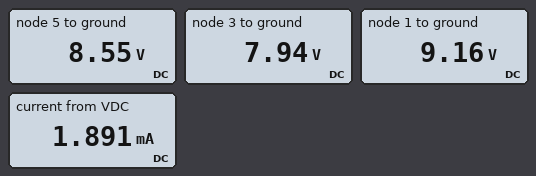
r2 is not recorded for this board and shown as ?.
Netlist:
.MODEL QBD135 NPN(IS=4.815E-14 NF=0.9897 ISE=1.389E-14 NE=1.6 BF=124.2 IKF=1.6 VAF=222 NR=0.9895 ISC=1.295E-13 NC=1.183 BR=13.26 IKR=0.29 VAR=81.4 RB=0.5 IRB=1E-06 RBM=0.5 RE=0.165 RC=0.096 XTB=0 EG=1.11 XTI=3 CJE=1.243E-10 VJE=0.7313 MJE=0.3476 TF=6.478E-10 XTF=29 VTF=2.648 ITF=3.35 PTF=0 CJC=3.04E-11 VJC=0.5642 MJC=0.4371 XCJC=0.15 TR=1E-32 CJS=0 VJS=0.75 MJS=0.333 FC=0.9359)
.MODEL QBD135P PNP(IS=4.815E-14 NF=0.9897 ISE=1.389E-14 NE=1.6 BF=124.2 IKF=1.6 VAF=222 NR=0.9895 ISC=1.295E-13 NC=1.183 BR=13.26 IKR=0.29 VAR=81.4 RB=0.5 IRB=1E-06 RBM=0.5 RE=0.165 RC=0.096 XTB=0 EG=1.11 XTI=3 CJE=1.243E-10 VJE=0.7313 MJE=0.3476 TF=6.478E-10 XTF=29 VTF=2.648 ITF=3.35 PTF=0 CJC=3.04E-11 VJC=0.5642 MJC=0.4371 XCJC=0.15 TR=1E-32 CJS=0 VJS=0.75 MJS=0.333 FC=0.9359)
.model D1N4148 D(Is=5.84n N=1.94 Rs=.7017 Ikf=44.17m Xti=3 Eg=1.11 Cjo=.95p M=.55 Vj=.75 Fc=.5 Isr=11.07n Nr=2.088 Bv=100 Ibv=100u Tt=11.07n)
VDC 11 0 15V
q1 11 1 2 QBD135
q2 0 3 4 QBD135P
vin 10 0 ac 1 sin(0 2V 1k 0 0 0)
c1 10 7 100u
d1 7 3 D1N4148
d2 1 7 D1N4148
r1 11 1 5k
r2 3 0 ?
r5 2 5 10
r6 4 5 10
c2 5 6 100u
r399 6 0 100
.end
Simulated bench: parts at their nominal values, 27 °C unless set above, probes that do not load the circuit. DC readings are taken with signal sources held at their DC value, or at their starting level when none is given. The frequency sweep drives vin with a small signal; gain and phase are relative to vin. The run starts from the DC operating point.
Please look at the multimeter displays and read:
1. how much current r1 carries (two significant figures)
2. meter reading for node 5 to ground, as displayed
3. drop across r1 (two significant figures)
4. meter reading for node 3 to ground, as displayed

1.2 mA
8.55 V
5.8 V
7.94 V
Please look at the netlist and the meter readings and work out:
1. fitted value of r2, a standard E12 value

6.8 kΩ
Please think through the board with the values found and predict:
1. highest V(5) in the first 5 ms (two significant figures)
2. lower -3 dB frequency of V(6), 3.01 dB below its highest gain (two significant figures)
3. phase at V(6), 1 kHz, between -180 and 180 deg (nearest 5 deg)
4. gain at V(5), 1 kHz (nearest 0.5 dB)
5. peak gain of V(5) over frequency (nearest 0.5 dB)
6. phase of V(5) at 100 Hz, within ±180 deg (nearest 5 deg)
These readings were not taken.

10 V
17 Hz
0 deg
-2.0 dB
-0.5 dB
0 deg
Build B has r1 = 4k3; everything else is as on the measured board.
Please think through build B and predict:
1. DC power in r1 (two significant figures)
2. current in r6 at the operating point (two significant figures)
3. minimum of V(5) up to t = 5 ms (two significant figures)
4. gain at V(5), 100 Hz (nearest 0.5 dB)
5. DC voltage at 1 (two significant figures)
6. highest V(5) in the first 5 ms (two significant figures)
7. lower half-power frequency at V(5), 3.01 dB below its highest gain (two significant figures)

6.6 mW
810 µA
7.3 V
-1.5 dB
9.7 V
11 V
570 mHz
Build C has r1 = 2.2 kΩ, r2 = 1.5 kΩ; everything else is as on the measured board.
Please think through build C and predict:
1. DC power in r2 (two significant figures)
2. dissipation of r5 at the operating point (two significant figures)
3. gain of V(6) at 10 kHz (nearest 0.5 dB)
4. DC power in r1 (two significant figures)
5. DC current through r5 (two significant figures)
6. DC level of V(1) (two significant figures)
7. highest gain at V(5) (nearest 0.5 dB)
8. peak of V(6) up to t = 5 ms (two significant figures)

20 mW
130 µW
-1.0 dB
30 mW
3.6 mA
6.9 V
-0.5 dB
1.8 V
